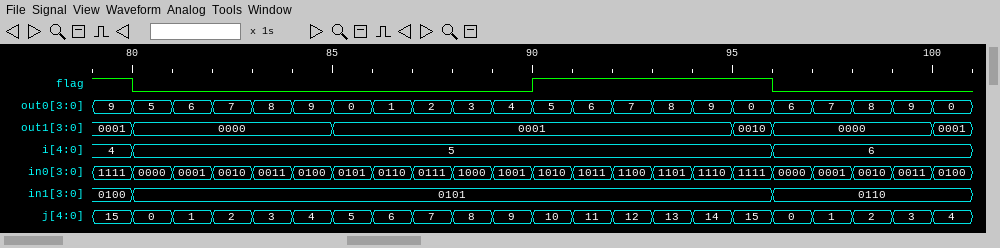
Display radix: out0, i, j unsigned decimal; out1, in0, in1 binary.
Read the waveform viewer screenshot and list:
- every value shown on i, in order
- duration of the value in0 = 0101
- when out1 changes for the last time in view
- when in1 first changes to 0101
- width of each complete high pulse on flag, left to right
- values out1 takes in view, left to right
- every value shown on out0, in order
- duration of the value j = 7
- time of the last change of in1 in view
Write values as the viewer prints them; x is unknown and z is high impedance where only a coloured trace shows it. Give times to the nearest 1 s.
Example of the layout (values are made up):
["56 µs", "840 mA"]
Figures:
["4, 5, 6", "1 s", "100 s", "80 s", "6 s", "0001, 0000, 0001, 0010, 0000, 0001", "9, 5, 6, 7, 8, 9, 0, 1, 2, 3, 4, 5, 6, 7, 8, 9, 0, 6, 7, 8, 9, 0", "1 s", "96 s"]
